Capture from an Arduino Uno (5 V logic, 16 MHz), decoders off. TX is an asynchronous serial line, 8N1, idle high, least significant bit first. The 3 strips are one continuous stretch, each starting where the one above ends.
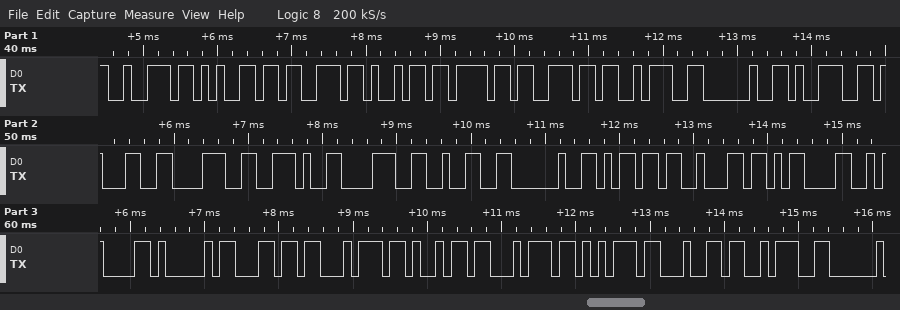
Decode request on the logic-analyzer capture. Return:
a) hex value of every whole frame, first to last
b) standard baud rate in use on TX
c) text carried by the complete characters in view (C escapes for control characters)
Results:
72 65 73 69 6F 6E 3A 20 39 31 38 2E 38 32 20 6D 62 0D 0A 41 6C 74 69 74 75 64 3A
9600 baud
"resion: 918.82 mb\r\nAltitud:"
